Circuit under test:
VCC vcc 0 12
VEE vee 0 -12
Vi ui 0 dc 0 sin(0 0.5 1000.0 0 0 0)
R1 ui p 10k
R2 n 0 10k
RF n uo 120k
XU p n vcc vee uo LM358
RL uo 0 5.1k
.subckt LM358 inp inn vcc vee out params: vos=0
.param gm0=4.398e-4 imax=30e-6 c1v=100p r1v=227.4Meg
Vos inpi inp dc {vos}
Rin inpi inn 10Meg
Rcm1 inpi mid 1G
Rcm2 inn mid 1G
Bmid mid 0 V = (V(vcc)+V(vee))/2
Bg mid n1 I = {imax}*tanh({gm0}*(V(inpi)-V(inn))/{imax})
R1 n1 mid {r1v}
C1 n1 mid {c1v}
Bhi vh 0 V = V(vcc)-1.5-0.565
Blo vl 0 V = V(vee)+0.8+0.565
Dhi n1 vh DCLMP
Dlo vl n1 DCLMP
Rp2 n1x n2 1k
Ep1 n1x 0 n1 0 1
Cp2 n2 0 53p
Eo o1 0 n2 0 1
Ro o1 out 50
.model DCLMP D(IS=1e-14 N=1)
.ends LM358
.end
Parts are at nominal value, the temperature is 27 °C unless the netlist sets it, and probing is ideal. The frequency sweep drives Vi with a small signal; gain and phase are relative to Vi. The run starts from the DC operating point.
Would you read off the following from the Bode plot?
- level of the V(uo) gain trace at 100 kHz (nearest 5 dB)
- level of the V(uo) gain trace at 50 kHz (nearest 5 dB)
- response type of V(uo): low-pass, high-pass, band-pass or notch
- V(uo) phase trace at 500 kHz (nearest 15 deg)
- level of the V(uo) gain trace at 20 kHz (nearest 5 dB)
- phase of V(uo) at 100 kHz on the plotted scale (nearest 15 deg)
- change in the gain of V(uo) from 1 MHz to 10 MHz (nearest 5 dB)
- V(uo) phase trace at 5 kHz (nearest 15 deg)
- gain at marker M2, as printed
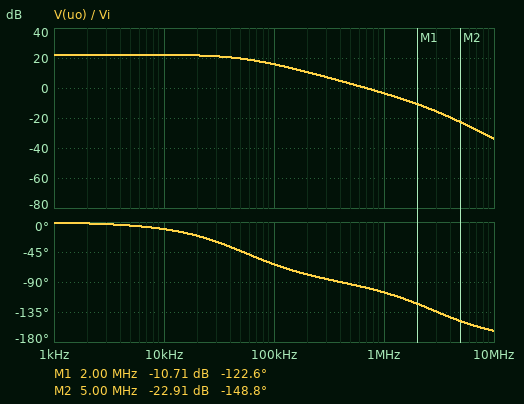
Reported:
15 dB
20 dB
low-pass
-90 deg
20 dB
-60 deg
-30 dB
0 deg
-22.91 dB
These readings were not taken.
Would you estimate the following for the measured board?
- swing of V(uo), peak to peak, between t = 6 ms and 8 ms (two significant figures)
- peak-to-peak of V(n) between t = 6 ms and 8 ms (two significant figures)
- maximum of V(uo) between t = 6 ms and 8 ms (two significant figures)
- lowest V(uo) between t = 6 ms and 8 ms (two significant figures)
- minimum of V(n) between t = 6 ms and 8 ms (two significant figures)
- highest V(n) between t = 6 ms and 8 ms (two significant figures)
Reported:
13 V
1.0 V
6.5 V
-6.5 V
-500 mV
500 mV
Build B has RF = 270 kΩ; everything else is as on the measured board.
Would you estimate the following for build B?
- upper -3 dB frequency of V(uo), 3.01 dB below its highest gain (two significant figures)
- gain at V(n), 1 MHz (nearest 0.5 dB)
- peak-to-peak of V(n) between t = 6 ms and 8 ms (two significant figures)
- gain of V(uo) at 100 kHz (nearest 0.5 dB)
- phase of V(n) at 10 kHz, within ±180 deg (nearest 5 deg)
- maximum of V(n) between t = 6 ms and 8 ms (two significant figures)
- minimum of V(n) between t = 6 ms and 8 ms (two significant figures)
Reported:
25 kHz
-32.5 dB
770 mV
16.5 dB
-20 deg
370 mV
-400 mV
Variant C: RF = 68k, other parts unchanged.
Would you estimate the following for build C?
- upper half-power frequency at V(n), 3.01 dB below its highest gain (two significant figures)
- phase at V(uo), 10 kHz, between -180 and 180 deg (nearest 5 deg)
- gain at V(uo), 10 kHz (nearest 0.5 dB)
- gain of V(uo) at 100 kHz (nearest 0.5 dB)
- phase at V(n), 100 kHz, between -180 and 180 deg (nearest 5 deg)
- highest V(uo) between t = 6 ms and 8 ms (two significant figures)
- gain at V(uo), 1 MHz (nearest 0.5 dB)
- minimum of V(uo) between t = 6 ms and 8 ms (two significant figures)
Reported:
91 kHz
-5 deg
18.0 dB
14.5 dB
-50 deg
3.9 V
-3.5 dB
-3.9 V
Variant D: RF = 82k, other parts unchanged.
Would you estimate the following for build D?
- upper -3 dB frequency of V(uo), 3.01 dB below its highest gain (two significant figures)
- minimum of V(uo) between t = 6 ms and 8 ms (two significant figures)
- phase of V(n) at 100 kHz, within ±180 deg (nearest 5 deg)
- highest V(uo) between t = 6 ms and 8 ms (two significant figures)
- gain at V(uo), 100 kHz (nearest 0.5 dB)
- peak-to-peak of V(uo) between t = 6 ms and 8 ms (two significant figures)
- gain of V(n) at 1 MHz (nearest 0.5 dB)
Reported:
77 kHz
-4.6 V
-55 deg
4.6 V
15.0 dB
9.2 V
-23.0 dB
